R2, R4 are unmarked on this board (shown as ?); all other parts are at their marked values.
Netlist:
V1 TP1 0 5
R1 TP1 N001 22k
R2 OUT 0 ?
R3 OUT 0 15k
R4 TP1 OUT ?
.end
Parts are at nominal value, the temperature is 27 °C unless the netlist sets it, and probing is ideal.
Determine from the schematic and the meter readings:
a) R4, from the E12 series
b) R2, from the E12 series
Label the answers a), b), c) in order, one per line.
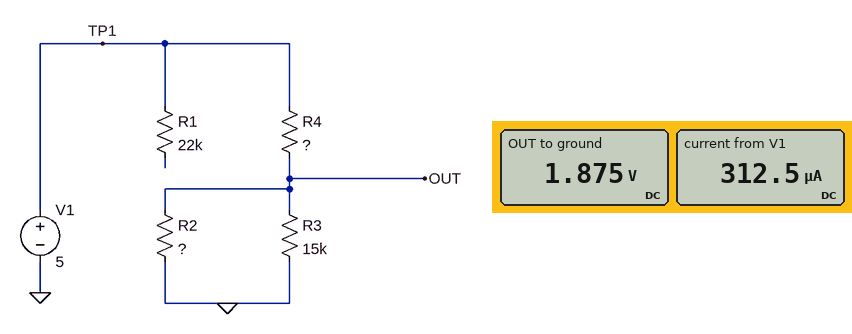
a) 10 kΩ
b) 10 kΩ
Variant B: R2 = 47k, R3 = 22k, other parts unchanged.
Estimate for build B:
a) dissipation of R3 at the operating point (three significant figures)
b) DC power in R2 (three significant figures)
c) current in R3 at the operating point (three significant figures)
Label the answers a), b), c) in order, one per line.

a) 409 µW
b) 191 µW
c) 136 µA
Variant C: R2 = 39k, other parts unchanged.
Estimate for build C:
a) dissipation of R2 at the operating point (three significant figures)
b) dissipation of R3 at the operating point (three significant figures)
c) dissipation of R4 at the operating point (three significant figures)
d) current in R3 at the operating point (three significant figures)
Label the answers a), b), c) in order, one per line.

a) 173 µW
b) 451 µW
c) 576 µW
d) 173 µA
